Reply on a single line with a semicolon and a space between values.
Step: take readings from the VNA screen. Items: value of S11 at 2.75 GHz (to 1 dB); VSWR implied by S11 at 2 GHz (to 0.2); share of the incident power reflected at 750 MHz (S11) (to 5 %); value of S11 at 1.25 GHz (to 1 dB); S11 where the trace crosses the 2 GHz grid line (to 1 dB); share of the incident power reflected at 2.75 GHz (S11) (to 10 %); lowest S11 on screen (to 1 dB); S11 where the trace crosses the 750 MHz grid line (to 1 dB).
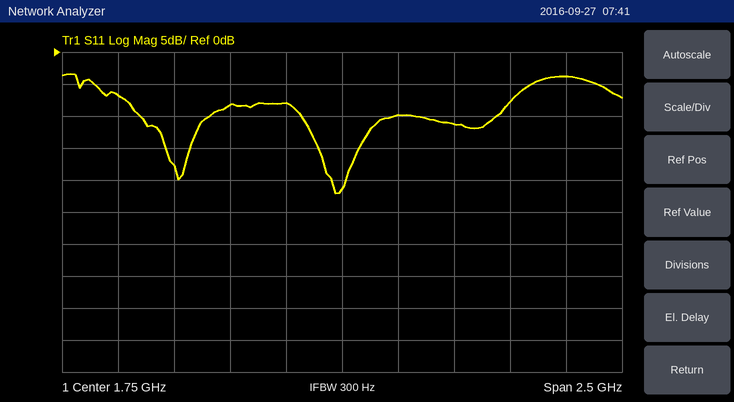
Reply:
-4 dB; 2.0; 20 %; -8 dB; -10 dB; 40 %; -22 dB; -7 dB
